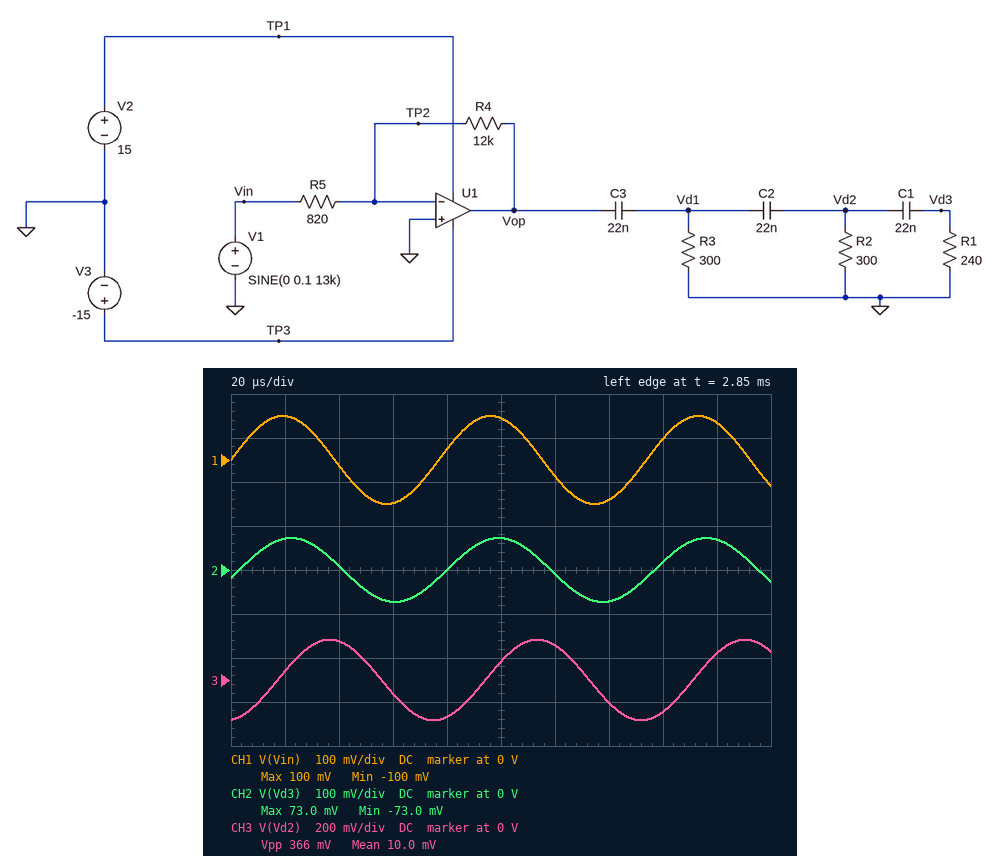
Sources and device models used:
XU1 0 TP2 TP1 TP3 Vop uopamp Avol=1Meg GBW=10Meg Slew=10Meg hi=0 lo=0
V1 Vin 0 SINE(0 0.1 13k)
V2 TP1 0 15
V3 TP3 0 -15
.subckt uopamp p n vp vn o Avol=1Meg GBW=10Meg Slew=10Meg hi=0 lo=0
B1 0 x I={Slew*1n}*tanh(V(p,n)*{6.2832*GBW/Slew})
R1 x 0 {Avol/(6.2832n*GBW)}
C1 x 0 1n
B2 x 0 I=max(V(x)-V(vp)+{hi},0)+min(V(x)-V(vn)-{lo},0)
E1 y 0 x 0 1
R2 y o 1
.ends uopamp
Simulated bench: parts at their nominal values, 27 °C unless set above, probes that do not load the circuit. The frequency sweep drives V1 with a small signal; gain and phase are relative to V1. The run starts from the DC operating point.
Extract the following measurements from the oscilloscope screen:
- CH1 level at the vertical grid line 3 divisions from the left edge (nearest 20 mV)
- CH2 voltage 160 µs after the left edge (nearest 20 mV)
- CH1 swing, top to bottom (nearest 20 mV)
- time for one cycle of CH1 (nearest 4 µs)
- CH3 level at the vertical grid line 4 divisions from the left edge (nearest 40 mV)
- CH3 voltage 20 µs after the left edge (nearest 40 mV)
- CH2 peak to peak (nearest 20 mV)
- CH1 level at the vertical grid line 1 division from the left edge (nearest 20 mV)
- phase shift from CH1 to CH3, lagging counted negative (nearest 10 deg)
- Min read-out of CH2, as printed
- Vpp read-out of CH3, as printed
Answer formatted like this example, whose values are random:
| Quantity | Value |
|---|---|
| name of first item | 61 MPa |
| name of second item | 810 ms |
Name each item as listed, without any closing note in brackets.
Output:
| Quantity | Value |
|---|---|
| CH1 level at the vertical grid line 3 divisions from the left edge | -100 mV |
| CH2 voltage 160 µs after the left edge | 20 mV |
| CH1 swing, top to bottom | 200 mV |
| time for one cycle of CH1 | 76 µs |
| CH3 level at the vertical grid line 4 divisions from the left edge | -160 mV |
| CH3 voltage 20 µs after the left edge | 40 mV |
| CH2 peak to peak | 140 mV |
| CH1 level at the vertical grid line 1 division from the left edge | 100 mV |
| phase shift from CH1 to CH3, lagging counted negative | -80 deg |
| Min read-out of CH2, as printed | -73.0 mV |
| Vpp read-out of CH3, as printed | 366 mV |
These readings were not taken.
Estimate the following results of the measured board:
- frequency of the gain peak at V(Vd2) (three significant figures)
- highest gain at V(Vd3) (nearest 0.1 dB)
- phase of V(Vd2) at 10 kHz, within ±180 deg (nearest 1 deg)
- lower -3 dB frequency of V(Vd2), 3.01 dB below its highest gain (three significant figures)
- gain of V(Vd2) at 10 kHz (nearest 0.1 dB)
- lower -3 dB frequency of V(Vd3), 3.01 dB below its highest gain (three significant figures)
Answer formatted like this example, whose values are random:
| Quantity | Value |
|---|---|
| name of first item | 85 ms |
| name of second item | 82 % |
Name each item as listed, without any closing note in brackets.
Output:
| Quantity | Value |
|---|---|
| frequency of the gain peak at V(Vd2) | 293 kHz |
| highest gain at V(Vd3) | 21.6 dB |
| phase of V(Vd2) at 10 kHz, within ±180 deg | -70 deg |
| lower -3 dB frequency of V(Vd2), 3.01 dB below its highest gain | 96.8 kHz |
| gain of V(Vd2) at 10 kHz | 2.7 dB |
| lower -3 dB frequency of V(Vd3), 3.01 dB below its highest gain | 103 kHz |
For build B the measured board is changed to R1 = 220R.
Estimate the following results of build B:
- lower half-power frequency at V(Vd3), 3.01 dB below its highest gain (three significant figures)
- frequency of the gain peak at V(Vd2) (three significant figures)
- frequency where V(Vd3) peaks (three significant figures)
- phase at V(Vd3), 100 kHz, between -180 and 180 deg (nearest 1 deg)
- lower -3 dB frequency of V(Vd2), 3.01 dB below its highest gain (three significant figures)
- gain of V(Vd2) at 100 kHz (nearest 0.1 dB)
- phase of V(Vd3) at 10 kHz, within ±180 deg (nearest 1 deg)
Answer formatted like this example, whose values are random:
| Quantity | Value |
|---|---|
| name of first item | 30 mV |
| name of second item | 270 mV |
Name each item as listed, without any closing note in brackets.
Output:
| Quantity | Value |
|---|---|
| lower half-power frequency at V(Vd3), 3.01 dB below its highest gain | 107 kHz |
| frequency of the gain peak at V(Vd2) | 300 kHz |
| frequency where V(Vd3) peaks | 306 kHz |
| phase at V(Vd3), 100 kHz, between -180 and 180 deg | -119 deg |
| lower -3 dB frequency of V(Vd2), 3.01 dB below its highest gain | 100 kHz |
| gain of V(Vd2) at 100 kHz | 18.5 dB |
| phase of V(Vd3) at 10 kHz, within ±180 deg | 2 deg |
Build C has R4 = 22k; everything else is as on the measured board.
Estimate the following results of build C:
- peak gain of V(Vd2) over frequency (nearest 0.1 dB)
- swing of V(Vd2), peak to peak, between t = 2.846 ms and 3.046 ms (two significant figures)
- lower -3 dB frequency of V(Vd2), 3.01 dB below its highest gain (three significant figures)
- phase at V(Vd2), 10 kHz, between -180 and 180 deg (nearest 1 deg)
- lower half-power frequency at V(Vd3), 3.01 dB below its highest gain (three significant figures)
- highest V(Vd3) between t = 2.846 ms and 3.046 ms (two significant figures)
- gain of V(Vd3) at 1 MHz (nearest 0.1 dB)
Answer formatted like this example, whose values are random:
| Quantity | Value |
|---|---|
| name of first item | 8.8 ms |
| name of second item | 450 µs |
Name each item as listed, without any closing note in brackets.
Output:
| Quantity | Value |
|---|---|
| peak gain of V(Vd2) over frequency | 25.8 dB |
| swing of V(Vd2), peak to peak, between t = 2.846 ms and 3.046 ms | 670 mV |
| lower -3 dB frequency of V(Vd2), 3.01 dB below its highest gain | 81.1 kHz |
| phase at V(Vd2), 10 kHz, between -180 and 180 deg | -71 deg |
| lower half-power frequency at V(Vd3), 3.01 dB below its highest gain | 87.6 kHz |
| highest V(Vd3) between t = 2.846 ms and 3.046 ms | 130 mV |
| gain of V(Vd3) at 1 MHz | 19.0 dB |
